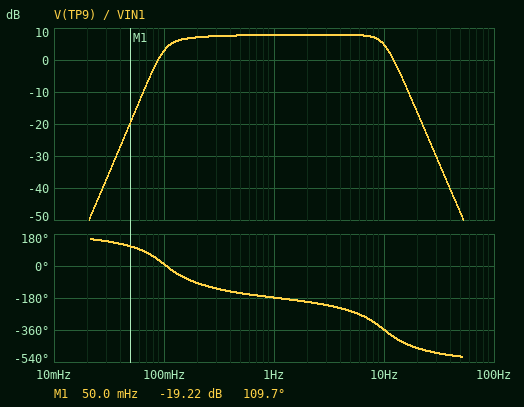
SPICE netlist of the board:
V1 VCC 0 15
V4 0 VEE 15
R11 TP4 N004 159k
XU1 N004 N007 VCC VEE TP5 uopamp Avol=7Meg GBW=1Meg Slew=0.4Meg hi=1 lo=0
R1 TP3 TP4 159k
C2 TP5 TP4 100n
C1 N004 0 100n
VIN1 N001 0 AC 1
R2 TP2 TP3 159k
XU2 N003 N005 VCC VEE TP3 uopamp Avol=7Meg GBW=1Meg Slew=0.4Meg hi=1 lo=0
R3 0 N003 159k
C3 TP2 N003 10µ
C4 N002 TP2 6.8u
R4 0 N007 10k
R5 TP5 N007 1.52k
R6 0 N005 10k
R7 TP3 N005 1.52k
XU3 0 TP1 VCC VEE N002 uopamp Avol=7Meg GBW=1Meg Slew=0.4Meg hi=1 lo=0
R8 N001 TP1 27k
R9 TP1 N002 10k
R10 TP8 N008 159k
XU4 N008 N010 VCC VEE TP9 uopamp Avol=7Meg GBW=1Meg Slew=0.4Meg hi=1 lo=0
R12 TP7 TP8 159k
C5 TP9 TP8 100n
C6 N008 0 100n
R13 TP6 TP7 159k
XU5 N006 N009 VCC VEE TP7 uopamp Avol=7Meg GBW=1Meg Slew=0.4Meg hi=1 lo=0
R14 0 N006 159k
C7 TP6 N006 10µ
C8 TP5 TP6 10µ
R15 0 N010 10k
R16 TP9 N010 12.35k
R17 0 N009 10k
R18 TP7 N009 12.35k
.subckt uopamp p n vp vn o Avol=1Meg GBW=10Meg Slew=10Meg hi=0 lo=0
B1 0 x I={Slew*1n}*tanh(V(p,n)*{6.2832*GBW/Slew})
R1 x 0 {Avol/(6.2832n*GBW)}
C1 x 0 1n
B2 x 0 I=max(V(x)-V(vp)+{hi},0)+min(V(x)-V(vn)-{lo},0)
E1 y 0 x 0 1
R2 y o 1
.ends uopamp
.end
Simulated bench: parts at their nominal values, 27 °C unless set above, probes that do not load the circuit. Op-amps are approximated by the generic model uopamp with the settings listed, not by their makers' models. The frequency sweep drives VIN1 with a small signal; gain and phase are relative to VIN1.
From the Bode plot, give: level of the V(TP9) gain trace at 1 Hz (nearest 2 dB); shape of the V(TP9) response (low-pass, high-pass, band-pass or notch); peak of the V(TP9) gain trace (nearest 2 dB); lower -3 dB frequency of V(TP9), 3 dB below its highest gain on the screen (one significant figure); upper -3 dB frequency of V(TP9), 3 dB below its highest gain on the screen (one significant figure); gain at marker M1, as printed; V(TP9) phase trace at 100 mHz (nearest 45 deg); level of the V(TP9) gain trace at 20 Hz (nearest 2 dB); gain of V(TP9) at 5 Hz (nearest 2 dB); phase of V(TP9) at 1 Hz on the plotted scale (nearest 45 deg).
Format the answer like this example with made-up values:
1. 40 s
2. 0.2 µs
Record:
1. 8 dB
2. band-pass
3. 8 dB
4. 100 mHz
5. 10 Hz
6. -19.22 dB
7. 0 deg
8. -16 dB
9. 8 dB
10. -180 deg
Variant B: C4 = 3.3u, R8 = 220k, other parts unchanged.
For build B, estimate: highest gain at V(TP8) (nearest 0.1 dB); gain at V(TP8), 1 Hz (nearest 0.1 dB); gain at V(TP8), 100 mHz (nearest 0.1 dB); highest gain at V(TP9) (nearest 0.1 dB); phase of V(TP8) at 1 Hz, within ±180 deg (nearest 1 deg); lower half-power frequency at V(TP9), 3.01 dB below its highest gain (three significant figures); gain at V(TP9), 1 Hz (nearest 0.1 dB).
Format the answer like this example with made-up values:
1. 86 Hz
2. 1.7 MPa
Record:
1. -15.9 dB
2. -17.6 dB
3. -27.4 dB
4. -10.4 dB
5. -165 deg
6. 228 mHz
7. -10.6 dB
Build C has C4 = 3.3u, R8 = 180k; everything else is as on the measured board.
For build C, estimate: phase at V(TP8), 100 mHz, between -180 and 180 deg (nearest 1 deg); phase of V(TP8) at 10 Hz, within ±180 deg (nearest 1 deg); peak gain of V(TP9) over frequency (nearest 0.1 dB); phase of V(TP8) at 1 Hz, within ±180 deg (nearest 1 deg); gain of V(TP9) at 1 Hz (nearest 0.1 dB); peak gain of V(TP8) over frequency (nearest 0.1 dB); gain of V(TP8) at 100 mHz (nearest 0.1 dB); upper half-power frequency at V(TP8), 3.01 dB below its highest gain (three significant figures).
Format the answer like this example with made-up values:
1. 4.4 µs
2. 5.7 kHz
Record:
1. 29 deg
2. 48 deg
3. -8.7 dB
4. -165 deg
5. -8.9 dB
6. -14.1 dB
7. -25.6 dB
8. 11.0 Hz
